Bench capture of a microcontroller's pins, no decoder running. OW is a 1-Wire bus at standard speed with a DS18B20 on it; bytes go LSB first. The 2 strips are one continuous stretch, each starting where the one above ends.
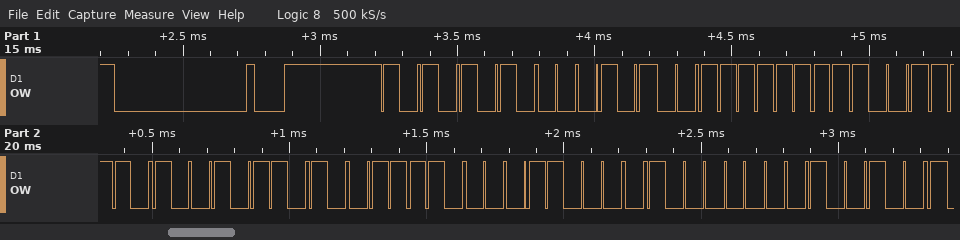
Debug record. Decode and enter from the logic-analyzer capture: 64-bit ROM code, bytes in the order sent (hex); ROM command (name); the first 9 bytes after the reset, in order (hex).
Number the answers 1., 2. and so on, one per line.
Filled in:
1. 28 FF 79 69 79 18 02 92
2. Match ROM
3. 55 28 FF 79 69 79 18 02 92
